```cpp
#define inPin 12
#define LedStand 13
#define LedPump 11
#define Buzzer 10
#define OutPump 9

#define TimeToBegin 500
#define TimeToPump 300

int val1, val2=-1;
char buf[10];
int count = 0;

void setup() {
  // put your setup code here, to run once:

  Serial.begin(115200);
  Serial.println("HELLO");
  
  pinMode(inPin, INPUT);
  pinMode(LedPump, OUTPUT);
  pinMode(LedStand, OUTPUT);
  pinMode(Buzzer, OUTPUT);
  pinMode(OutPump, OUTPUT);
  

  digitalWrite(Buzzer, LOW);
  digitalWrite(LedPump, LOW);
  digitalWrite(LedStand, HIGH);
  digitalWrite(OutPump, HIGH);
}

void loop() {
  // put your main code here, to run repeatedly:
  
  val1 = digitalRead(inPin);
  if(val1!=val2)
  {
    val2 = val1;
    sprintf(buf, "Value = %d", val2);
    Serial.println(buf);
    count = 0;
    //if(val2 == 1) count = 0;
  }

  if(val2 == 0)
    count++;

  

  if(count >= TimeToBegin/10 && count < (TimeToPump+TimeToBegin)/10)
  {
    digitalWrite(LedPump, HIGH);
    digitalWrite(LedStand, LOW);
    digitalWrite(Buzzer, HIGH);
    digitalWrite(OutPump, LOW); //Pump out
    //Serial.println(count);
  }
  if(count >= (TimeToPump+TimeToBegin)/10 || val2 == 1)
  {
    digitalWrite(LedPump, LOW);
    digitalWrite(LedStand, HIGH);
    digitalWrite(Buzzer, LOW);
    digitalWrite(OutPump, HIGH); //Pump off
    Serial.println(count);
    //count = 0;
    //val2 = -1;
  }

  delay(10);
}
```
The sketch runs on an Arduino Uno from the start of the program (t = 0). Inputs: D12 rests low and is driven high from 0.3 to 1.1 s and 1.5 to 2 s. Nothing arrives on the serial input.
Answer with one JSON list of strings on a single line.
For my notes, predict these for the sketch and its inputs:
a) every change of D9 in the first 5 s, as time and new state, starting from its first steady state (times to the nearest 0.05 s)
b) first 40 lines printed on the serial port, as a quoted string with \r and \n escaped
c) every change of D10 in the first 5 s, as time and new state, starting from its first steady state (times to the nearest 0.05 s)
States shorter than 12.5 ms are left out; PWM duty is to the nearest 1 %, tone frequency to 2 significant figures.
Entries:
["0 s high; 2.5 s low; 2.8 s high", "\"HELLO\\r\\nValue = 0\\r\\nValue = 1\\r\\n0\\r\\n0\\r\\n0\\r\\n0\\r\\n0\\r\\n0\\r\\n0\\r\\n0\\r\\n0\\r\\n0\\r\\n0\\r\\n0\\r\\n0\\r\\n0\\r\\n0\\r\\n0\\r\\n0\\r\\n0\\r\\n0\\r\\n0\\r\\n0\\r\\n0\\r\\n0\\r\\n0\\r\\n0\\r\\n0\\r\\n0\\r\\n0\\r\\n0\\r\\n0\\r\\n0\\r\\n0\\r\\n0\\r\\n0\\r\\n0\\r\\n0\\r\\n0\\r\\n\"", "0 s low; 2.5 s high; 2.8 s low"]
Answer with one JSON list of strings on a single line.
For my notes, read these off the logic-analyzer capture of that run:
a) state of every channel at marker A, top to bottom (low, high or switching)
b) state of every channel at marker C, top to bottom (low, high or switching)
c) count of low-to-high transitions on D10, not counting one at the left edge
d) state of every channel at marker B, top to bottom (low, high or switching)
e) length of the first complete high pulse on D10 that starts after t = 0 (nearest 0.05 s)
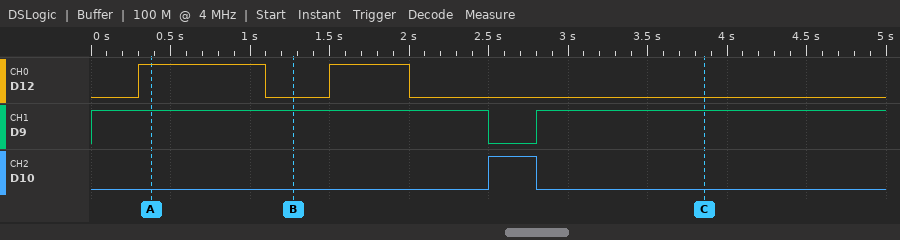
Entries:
["D12 high, D9 high, D10 low", "D12 low, D9 high, D10 low", "1", "D12 low, D9 high, D10 low", "0.30 s"]
